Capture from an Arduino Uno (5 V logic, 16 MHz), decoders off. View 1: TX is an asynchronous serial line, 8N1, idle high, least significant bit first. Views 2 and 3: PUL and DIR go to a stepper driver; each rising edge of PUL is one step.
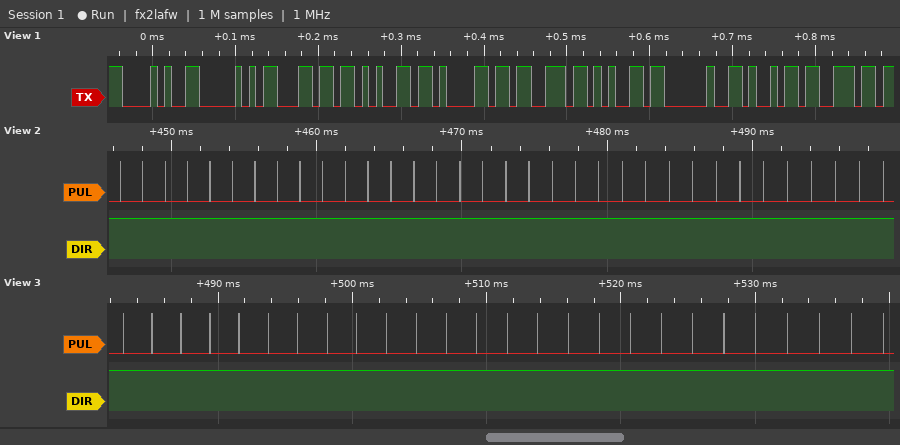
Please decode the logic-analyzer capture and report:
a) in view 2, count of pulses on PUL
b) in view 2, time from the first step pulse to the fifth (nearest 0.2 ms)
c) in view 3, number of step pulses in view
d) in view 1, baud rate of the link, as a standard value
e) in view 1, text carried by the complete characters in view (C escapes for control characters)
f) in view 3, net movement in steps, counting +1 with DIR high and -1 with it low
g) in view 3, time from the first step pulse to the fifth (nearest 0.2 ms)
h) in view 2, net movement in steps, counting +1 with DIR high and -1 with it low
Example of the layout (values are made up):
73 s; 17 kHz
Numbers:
34; 6.2 ms; 26; 115200 baud; "(Please in"; +26; 8.6 ms; +34
